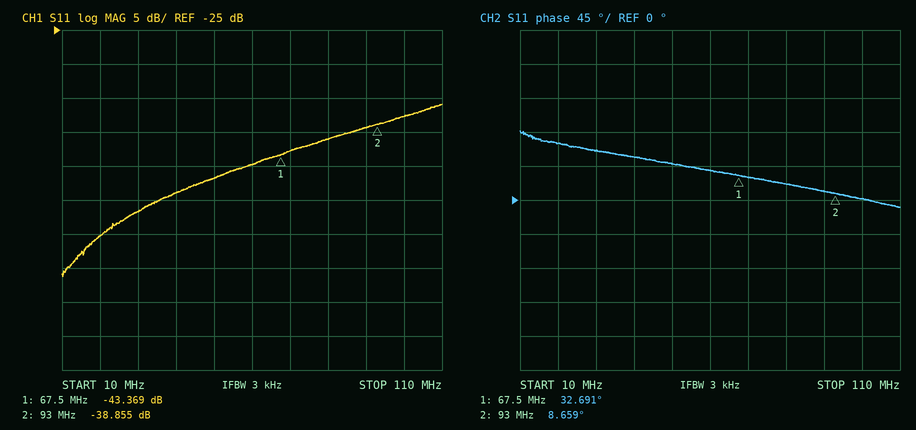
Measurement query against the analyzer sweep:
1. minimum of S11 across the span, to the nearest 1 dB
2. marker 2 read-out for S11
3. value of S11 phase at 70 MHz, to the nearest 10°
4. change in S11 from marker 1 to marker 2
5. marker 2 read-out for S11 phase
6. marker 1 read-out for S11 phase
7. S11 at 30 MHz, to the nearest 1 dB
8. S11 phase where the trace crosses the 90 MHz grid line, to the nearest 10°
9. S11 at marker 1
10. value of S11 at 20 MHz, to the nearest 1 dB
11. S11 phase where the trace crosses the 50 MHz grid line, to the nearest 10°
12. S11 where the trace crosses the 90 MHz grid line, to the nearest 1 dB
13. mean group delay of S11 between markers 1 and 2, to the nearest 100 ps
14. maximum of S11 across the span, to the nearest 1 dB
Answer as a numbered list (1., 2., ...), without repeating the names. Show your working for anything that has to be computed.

1. -61 dB
2. -38.855 dB
3. 30°
4. -38.855 − (-43.369) = 4.514 dB
5. 8.659°
6. 32.691°
7. -52 dB
8. 10°
9. -43.369 dB
10. -55 dB
11. 50°
12. -39 dB
13. −(8.659° − (32.691°))/(360° × 25.5 MHz) ≈ 2.6 ns
14. -36 dB
